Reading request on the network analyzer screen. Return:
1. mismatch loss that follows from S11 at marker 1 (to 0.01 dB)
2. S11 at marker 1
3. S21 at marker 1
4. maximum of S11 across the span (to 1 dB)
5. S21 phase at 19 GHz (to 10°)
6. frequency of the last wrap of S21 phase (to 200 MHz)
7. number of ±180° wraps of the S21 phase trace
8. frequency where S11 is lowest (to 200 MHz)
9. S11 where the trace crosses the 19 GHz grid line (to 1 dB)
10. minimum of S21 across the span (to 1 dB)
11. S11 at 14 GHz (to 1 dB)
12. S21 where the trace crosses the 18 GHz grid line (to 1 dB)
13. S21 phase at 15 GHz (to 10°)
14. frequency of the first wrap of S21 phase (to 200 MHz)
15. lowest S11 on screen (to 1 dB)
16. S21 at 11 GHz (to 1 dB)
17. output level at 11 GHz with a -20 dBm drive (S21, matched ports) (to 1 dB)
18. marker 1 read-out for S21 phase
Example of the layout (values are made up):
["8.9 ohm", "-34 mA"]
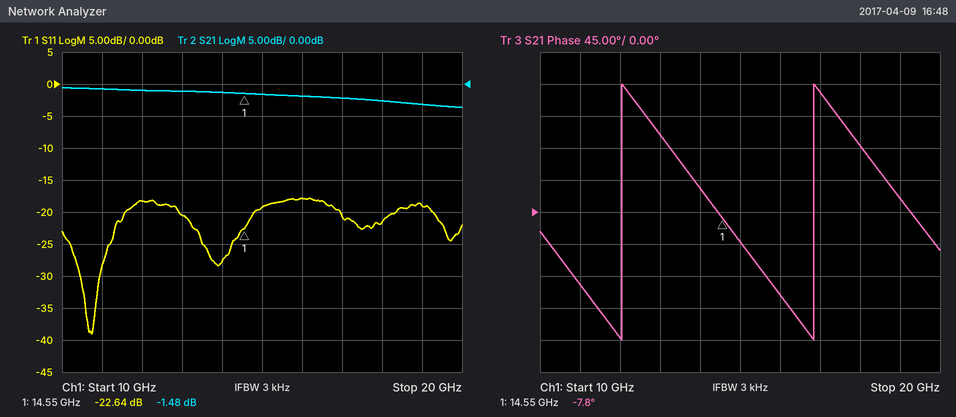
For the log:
["0.02 dB", "-22.64 dB", "-1.48 dB", "-18 dB", "20°", "16.8 GHz", "2", "10.8 GHz", "-19 dB", "-4 dB", "-28 dB", "-3 dB", "-40°", "12.0 GHz", "-39 dB", "-1 dB", "-21 dBm", "-7.8°"]
